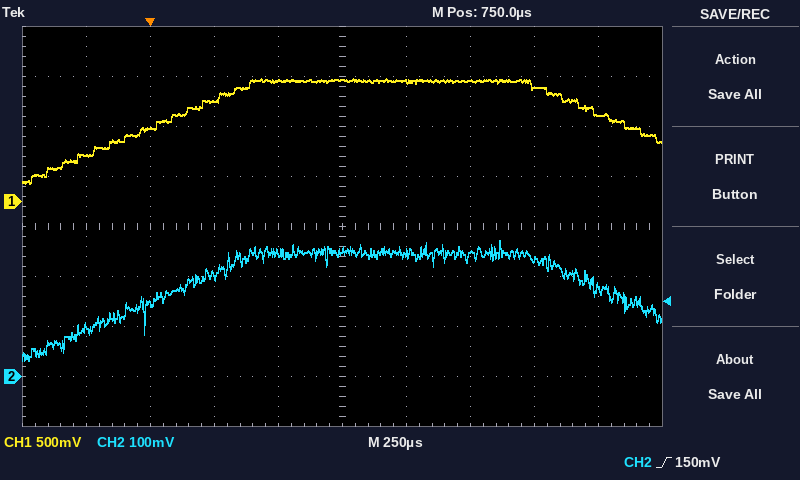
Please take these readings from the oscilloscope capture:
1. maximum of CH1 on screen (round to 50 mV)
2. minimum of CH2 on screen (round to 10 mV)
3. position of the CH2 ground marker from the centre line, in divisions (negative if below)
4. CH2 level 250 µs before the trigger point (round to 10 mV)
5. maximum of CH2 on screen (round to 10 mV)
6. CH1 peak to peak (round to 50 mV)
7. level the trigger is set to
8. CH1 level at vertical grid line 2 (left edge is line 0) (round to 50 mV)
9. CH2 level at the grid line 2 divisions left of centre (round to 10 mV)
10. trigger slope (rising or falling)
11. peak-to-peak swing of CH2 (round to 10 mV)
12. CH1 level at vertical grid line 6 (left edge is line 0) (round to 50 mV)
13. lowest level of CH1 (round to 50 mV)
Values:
1.25 V
30 mV
-3.0 div
100 mV
270 mV
1.05 V
150 mV
750 mV
200 mV
rising
240 mV
1.20 V
200 mV
